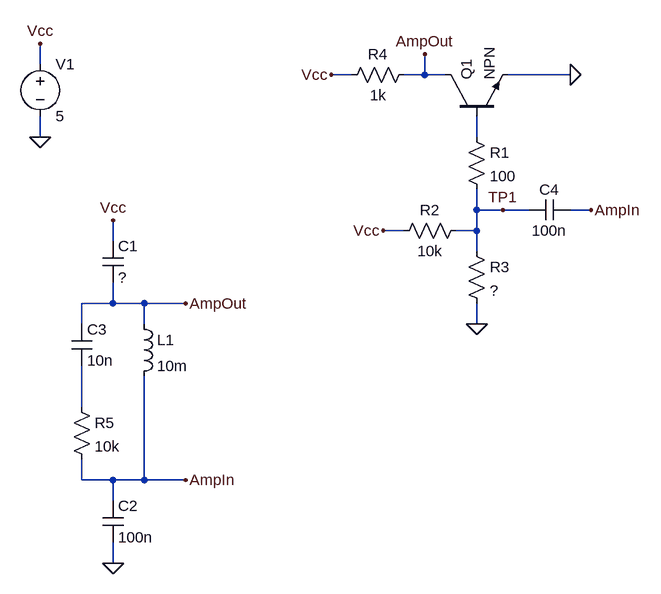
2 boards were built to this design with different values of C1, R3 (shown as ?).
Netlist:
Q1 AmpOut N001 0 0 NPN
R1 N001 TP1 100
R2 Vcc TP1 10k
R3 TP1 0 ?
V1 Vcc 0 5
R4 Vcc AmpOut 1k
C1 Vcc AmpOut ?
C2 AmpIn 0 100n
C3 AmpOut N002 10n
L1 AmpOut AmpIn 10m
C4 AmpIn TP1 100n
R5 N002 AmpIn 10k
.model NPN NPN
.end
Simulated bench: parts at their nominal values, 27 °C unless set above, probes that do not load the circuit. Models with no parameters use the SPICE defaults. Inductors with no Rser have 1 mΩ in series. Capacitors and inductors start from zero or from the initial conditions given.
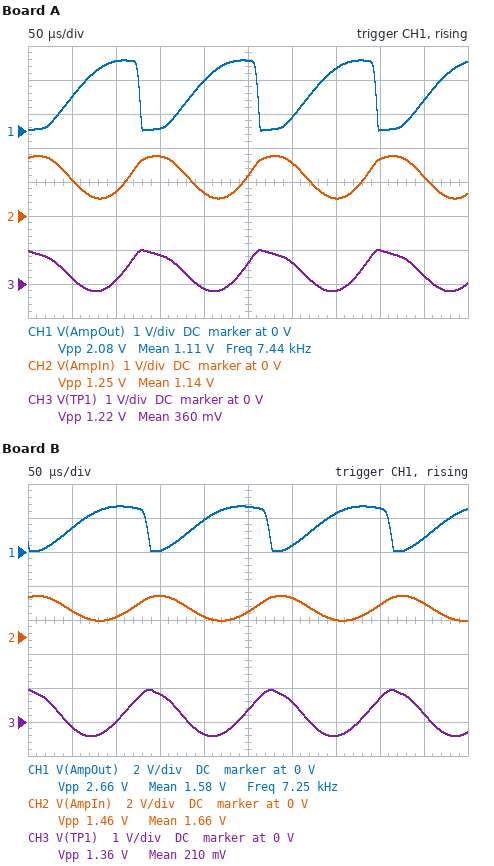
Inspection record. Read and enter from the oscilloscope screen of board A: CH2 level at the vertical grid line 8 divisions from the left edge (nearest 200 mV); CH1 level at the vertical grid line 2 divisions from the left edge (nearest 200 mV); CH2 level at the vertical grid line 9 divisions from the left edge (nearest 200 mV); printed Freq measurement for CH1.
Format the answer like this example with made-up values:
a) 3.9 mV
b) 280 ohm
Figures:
a) 1.6 V
b) 2.0 V
c) 1.2 V
d) 7.44 kHz
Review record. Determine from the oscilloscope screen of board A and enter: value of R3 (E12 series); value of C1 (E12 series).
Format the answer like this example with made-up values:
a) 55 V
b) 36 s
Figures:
a) 1.5 kΩ
b) 220 nF
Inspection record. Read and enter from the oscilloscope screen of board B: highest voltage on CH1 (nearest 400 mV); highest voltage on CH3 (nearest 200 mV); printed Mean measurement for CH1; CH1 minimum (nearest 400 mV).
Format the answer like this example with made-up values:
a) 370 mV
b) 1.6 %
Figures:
a) 2.8 V
b) 1.0 V
c) 1.58 V
d) 0 V
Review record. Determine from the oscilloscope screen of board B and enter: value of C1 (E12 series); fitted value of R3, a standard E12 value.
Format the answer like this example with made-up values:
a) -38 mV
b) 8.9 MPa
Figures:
a) 180 nF
b) 560 Ω
